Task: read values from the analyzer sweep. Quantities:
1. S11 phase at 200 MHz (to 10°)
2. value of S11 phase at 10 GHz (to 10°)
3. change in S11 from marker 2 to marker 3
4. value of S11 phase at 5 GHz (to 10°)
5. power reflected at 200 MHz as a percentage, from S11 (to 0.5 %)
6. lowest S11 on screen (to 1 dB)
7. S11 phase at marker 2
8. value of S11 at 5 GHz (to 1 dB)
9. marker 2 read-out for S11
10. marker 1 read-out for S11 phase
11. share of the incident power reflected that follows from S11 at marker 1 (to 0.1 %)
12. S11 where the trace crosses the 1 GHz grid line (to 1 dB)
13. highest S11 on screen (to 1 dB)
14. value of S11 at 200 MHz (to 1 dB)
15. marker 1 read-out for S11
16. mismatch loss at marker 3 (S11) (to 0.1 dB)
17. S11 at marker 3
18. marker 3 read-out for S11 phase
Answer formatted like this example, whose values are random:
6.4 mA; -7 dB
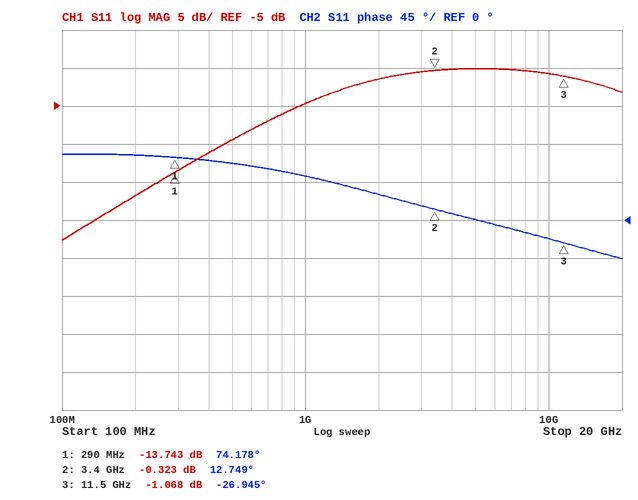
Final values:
80°; -20°; -0.745 dB; 0°; 2.0 %; -23 dB; 12.749°; 0 dB; -0.323 dB; 74.178°; 4.2 %; -5 dB; 0 dB; -17 dB; -13.743 dB; 6.6 dB; -1.068 dB; -26.945°
